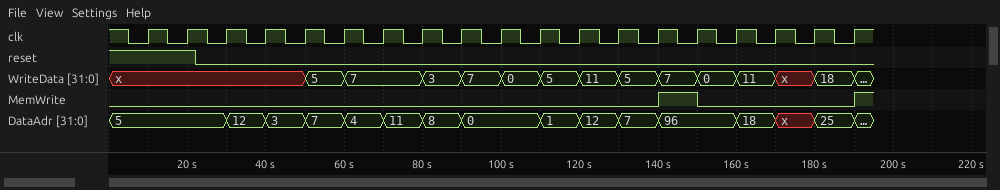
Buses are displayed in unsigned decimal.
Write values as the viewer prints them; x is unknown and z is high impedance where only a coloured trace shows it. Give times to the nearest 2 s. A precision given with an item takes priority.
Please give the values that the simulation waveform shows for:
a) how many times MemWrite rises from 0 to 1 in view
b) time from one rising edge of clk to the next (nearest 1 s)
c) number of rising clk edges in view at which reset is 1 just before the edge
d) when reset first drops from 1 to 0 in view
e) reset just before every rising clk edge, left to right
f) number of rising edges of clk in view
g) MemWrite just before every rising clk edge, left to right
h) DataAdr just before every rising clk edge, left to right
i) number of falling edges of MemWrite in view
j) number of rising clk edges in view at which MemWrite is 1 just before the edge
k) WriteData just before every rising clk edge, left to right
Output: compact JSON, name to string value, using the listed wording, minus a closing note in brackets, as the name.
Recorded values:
{"how many times MemWrite rises from 0 to 1 in view": "2", "time from one rising edge of clk to the next": "10 s", "number of rising clk edges in view at which reset is 1 just before the edge": "2", "when reset first drops from 1 to 0 in view": "22 s", "reset just before every rising clk edge, left to right": "1 1 0 0 0 0 0 0 0 0 0 0 0 0 0 0 0 0 0", "number of rising edges of clk in view": "19", "MemWrite just before every rising clk edge, left to right": "0 0 0 0 0 0 0 0 0 0 0 0 0 0 1 0 0 0 0", "DataAdr just before every rising clk edge, left to right": "5, 5, 5, 12, 3, 7, 4, 11, 8, 0, 0, 1, 12, 7, 96, 96, 18, x, 25", "number of falling edges of MemWrite in view": "1", "number of rising clk edges in view at which MemWrite is 1 just before the edge": "1", "WriteData just before every rising clk edge, left to right": "x, x, x, x, x, 5, 7, 7, 3, 7, 0, 5, 11, 5, 7, 0, 11, x, 18"}
